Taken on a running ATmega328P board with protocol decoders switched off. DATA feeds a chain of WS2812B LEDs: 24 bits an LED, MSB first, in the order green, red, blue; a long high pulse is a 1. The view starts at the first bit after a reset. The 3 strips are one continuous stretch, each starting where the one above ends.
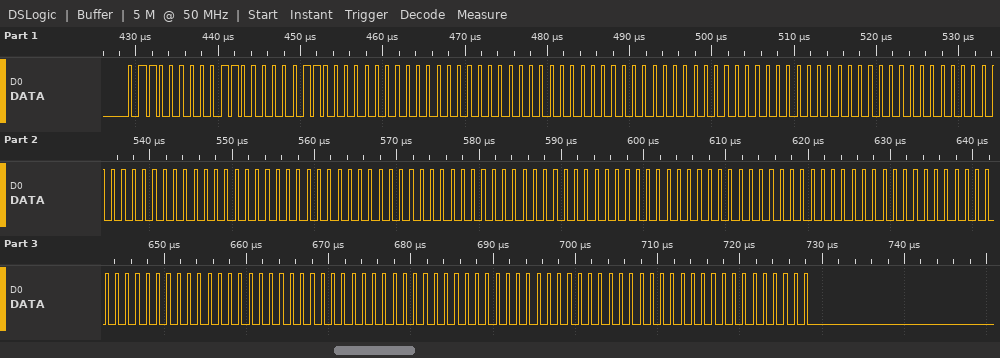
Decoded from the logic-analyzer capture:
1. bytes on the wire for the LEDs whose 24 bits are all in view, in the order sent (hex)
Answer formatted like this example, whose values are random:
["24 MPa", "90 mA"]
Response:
["60 60 60 00 00 00 00 00 00 00 00 00 00 00 00 00 00 00 00 00 00 00 00 00 00 00 00 00 00 00"]
